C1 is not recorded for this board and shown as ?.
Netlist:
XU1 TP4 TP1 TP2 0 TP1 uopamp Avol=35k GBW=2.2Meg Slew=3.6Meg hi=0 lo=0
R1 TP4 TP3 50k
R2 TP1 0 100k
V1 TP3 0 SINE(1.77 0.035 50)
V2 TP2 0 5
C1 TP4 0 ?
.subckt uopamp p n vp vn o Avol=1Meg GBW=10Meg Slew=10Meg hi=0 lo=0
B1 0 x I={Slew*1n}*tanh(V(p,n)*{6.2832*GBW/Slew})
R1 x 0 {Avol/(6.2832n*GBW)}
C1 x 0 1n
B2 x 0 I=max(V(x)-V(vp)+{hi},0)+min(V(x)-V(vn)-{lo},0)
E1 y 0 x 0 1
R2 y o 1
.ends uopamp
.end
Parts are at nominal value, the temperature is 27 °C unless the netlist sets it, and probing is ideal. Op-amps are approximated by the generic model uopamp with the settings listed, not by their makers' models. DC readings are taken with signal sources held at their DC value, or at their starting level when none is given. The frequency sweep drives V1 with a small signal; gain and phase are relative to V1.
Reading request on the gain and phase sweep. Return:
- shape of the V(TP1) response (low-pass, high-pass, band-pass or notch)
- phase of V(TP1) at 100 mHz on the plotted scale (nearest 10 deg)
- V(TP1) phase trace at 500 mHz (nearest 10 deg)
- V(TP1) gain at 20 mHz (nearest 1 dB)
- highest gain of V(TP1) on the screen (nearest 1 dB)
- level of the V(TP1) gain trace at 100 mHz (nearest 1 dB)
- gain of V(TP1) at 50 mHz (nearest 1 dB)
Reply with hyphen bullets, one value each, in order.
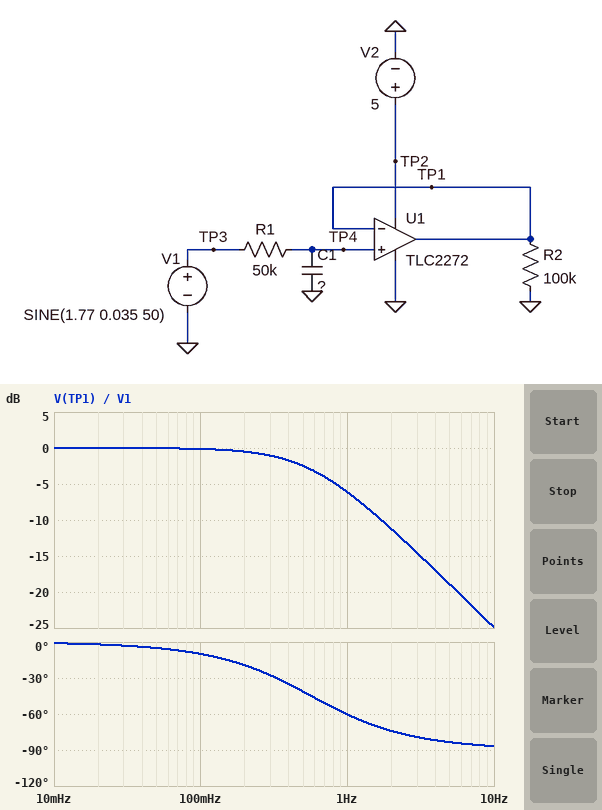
- low-pass
- -10 deg
- -40 deg
- 0 dB
- 0 dB
- 0 dB
- 0 dB
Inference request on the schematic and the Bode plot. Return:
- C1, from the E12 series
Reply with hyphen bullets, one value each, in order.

- 5.6 µF
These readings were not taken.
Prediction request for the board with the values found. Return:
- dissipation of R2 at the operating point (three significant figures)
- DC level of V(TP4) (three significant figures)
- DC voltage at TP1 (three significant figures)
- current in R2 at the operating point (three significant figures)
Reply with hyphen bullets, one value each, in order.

- 31.3 µW
- 1.77 V
- 1.77 V
- 17.7 µA
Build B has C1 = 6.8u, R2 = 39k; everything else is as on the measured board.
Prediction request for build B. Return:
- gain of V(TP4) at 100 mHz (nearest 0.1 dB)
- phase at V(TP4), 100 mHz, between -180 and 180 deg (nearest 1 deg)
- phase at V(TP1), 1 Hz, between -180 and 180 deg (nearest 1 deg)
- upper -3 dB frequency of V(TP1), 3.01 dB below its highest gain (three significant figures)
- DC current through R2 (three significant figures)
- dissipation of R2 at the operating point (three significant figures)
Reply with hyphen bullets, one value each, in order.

- -0.2 dB
- -12 deg
- -65 deg
- 468 mHz
- 45.4 µA
- 80.3 µW
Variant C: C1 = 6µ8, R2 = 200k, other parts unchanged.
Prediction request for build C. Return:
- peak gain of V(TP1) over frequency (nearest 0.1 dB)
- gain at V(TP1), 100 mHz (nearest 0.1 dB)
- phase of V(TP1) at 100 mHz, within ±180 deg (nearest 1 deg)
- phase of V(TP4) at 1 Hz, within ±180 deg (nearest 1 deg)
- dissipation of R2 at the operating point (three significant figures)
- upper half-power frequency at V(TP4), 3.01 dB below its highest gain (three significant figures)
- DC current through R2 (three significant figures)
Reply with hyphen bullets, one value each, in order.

- 0 dB
- -0.2 dB
- -12 deg
- -65 deg
- 15.7 µW
- 468 mHz
- 8.85 µA
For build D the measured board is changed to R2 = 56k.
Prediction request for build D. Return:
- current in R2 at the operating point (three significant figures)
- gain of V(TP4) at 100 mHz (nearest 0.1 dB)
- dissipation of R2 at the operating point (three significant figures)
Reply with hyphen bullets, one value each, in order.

- 31.6 µA
- -0.1 dB
- 55.9 µW
